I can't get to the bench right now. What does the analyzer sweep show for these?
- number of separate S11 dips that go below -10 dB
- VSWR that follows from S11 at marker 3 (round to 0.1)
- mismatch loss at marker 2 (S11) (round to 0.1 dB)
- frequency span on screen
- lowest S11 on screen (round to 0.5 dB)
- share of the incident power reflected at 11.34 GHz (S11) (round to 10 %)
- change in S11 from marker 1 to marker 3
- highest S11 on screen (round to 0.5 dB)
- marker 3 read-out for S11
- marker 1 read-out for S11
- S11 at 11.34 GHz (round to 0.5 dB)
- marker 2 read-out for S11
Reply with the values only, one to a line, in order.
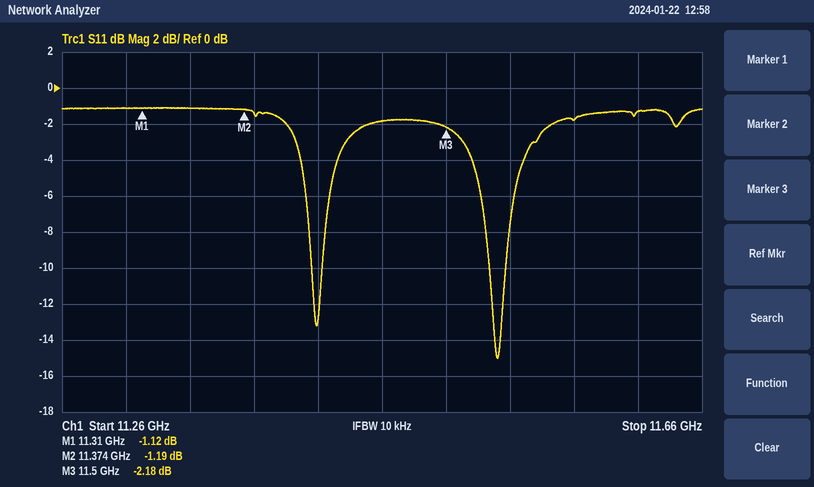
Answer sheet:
2
8.0
6.2 dB
400 MHz
-15.0 dB
80 %
-1.06 dB
-1.0 dB
-2.18 dB
-1.12 dB
-1.0 dB
-1.19 dB
